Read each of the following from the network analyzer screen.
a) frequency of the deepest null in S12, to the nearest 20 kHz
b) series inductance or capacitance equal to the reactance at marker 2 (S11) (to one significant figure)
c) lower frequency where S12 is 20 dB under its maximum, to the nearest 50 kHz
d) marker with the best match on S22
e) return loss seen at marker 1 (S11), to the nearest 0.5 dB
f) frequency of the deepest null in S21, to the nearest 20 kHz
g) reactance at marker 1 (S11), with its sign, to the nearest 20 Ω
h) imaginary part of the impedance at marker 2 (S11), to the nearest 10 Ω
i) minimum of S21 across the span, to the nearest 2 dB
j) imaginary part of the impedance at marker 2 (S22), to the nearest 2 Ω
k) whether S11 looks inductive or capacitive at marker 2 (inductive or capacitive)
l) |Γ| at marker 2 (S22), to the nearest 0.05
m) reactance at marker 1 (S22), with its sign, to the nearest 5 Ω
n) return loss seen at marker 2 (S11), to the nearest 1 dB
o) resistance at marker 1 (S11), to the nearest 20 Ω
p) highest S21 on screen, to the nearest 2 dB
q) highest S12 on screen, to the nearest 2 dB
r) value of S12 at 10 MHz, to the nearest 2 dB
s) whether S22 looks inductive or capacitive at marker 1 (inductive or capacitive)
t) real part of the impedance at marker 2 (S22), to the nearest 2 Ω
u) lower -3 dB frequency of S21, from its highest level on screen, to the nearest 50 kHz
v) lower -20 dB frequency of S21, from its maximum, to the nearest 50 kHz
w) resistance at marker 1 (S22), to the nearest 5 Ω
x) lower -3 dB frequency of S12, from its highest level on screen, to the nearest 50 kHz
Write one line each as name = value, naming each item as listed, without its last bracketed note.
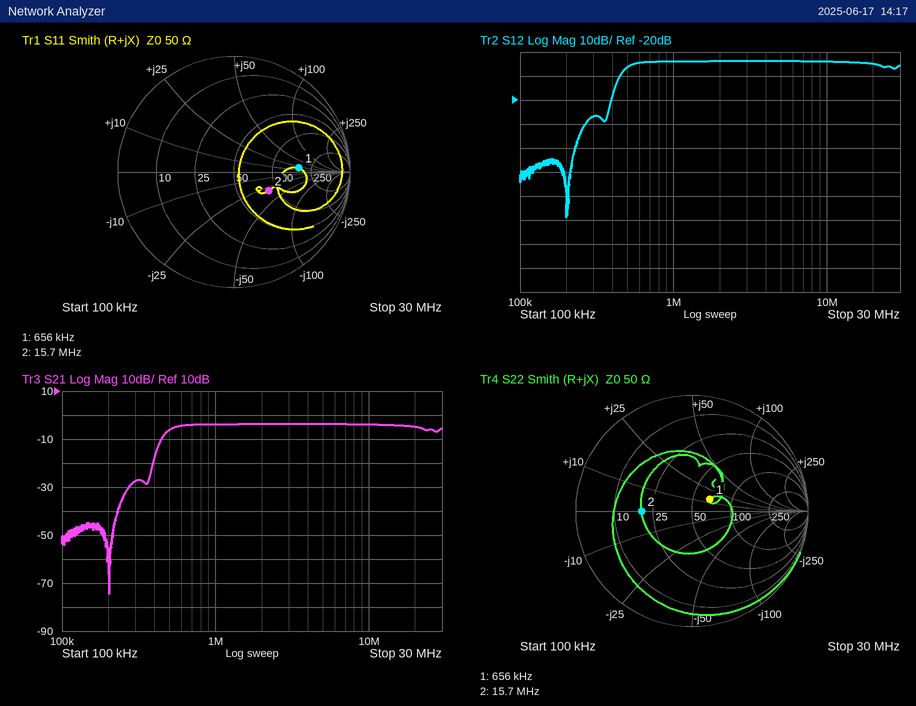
frequency of the deepest null in S12, to the nearest 20 kHz = 200 kHz
series inductance or capacitance equal to the reactance at marker 2 (S11) = 300 pF
lower frequency where S12 is 20 dB under its maximum, to the nearest 50 kHz = 400 kHz
marker with the best match on S22 = marker 1
return loss seen at marker 1 (S11), to the nearest 0.5 dB = 5.0 dB
frequency of the deepest null in S21, to the nearest 20 kHz = 200 kHz
reactance at marker 1 (S11), with its sign, to the nearest 20 Ω = +20 Ω
imaginary part of the impedance at marker 2 (S11), to the nearest 10 Ω = -30 Ω
minimum of S21 across the span, to the nearest 2 dB = -74 dB
imaginary part of the impedance at marker 2 (S22), to the nearest 2 Ω = 0 Ω
whether S11 looks inductive or capacitive at marker 2 = capacitive
|Γ| at marker 2 (S22), to the nearest 0.05 = 0.45
reactance at marker 1 (S22), with its sign, to the nearest 5 Ω = +15 Ω
return loss seen at marker 2 (S11), to the nearest 1 dB = 9 dB
resistance at marker 1 (S11), to the nearest 20 Ω = 180 Ω
highest S21 on screen, to the nearest 2 dB = -4 dB
highest S12 on screen, to the nearest 2 dB = -4 dB
value of S12 at 10 MHz, to the nearest 2 dB = -4 dB
whether S22 looks inductive or capacitive at marker 1 = inductive
real part of the impedance at marker 2 (S22), to the nearest 2 Ω = 20 Ω
lower -3 dB frequency of S21, from its highest level on screen, to the nearest 50 kHz = 500 kHz
lower -20 dB frequency of S21, from its maximum, to the nearest 50 kHz = 400 kHz
resistance at marker 1 (S22), to the nearest 5 Ω = 65 Ω
lower -3 dB frequency of S12, from its highest level on screen, to the nearest 50 kHz = 500 kHz
